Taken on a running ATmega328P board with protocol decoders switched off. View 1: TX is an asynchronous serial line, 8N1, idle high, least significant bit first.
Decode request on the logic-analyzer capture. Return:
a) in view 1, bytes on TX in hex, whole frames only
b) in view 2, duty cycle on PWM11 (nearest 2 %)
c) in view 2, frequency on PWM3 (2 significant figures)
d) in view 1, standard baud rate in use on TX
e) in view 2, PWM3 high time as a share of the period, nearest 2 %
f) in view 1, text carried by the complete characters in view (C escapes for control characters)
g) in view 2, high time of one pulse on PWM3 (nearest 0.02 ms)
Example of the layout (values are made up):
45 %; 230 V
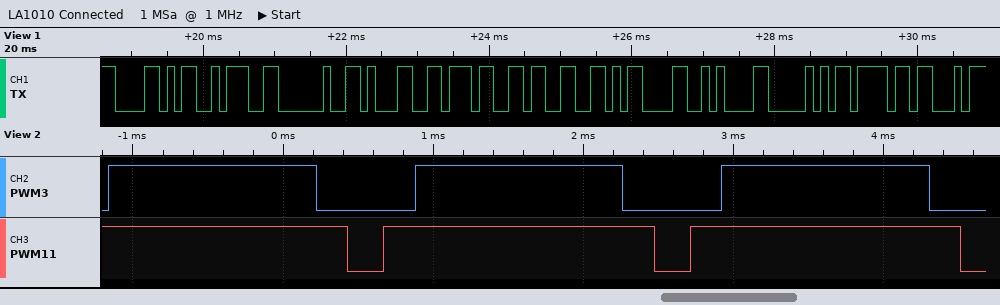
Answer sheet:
58 3A 20 31 37 33 0D 0A 50 6F; 88 %; 490 Hz; 9600 baud; 68 %; "X: 173\r\nPo"; 1.38 ms
